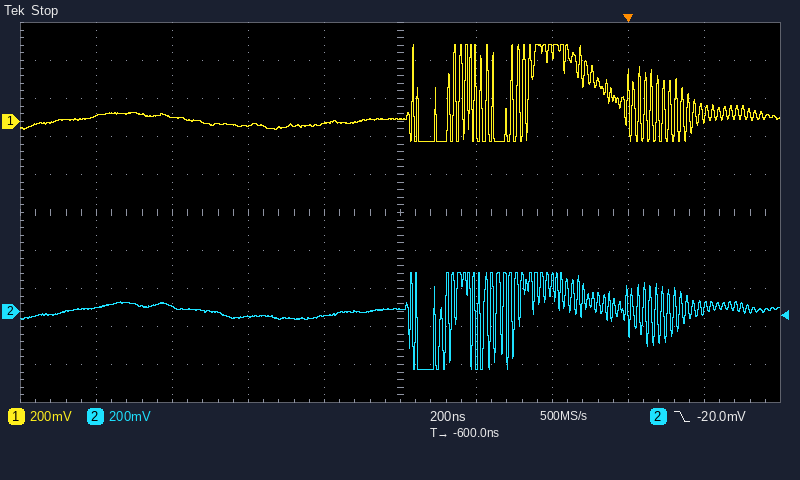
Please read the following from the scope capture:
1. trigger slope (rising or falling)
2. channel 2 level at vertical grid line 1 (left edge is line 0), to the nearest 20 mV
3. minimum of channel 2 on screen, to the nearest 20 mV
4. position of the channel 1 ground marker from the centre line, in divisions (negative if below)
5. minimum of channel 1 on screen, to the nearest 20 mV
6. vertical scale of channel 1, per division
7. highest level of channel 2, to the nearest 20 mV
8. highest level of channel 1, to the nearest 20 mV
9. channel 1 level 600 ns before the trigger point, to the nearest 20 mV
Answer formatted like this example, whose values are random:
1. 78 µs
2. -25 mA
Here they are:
1. falling
2. 20 mV
3. -300 mV
4. +2.4 div
5. -100 mV
6. 200 mV
7. 200 mV
8. 400 mV
9. 20 mV
